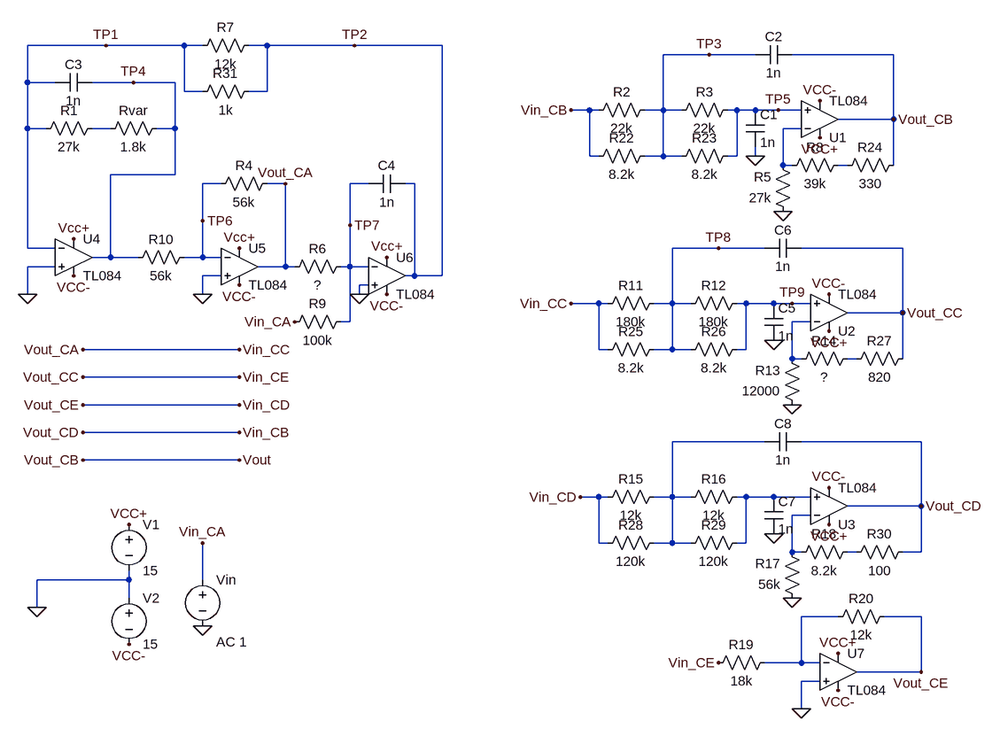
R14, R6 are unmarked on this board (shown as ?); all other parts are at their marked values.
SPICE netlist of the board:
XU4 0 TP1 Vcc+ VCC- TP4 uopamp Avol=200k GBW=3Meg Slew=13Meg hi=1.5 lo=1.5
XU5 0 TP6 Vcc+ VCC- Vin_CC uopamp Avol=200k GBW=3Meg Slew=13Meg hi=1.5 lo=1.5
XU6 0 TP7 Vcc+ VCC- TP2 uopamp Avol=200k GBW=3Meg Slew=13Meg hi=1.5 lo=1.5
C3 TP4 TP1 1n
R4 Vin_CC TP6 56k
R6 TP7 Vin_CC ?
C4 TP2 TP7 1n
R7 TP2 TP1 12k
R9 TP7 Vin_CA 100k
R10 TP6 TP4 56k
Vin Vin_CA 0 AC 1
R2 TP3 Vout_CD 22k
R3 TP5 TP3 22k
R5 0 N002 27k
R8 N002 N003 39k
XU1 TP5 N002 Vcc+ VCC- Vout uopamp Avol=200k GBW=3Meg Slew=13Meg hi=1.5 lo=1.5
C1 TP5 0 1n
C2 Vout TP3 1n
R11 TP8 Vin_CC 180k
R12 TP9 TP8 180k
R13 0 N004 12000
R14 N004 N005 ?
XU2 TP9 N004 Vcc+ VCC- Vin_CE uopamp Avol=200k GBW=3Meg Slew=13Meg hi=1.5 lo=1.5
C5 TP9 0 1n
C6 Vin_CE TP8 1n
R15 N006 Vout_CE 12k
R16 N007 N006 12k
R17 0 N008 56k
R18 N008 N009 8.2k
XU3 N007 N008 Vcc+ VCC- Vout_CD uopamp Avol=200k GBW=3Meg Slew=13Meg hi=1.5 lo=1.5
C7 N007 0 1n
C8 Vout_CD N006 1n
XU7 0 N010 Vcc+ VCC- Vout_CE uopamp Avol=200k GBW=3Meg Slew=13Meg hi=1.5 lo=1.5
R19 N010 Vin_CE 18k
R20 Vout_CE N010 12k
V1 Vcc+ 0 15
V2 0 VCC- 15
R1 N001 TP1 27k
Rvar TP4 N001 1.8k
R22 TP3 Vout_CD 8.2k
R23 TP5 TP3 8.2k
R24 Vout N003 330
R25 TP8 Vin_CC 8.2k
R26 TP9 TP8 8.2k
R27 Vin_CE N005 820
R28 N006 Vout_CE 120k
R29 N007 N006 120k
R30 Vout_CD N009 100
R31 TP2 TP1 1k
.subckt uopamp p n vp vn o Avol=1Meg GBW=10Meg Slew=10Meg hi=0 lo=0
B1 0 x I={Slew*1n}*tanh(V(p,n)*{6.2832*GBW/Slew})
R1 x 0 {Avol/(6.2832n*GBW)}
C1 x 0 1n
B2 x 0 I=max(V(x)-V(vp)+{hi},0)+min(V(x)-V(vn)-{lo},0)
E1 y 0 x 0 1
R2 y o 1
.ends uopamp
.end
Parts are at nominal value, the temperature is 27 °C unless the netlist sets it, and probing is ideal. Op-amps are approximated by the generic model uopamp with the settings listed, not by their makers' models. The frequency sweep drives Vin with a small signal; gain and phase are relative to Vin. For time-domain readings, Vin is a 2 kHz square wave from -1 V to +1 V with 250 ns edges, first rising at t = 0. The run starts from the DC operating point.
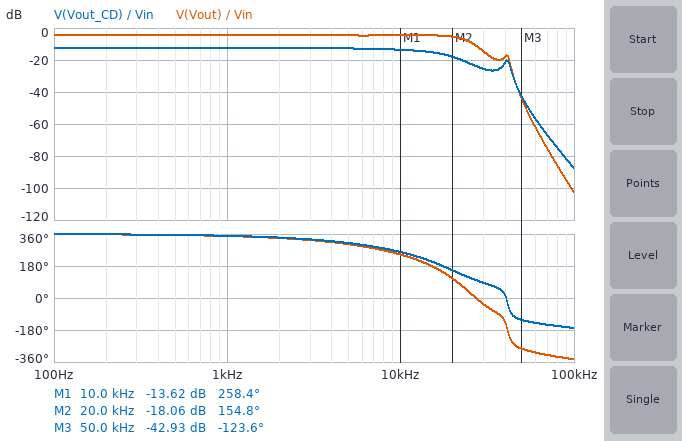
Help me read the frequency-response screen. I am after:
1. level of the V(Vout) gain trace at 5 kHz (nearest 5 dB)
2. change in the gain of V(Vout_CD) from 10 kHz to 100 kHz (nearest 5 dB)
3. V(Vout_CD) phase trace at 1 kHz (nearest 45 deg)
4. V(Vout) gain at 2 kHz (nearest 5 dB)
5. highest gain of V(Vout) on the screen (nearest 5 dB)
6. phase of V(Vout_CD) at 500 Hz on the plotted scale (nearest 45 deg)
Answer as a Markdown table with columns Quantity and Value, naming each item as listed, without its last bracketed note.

| Quantity | Value |
|---|---|
| level of the V(Vout) gain trace at 5 kHz | -5 dB |
| change in the gain of V(Vout_CD) from 10 kHz to 100 kHz | -75 dB |
| V(Vout_CD) phase trace at 1 kHz | 360 deg |
| V(Vout) gain at 2 kHz | -5 dB |
| highest gain of V(Vout) on the screen | -5 dB |
| phase of V(Vout_CD) at 500 Hz on the plotted scale | 360 deg |
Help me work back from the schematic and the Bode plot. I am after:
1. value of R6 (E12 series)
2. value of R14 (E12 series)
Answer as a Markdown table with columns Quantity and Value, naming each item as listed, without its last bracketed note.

| Quantity | Value |
|---|---|
| value of R6 | 15 kΩ |
| value of R14 | 12 kΩ |
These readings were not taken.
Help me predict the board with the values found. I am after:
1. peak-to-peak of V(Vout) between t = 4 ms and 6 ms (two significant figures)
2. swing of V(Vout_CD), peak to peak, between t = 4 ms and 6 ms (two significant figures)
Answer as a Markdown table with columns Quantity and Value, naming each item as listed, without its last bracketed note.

| Quantity | Value |
|---|---|
| peak-to-peak of V(Vout) between t = 4 ms and 6 ms | 1.5 V |
| swing of V(Vout_CD), peak to peak, between t = 4 ms and 6 ms | 510 mV |
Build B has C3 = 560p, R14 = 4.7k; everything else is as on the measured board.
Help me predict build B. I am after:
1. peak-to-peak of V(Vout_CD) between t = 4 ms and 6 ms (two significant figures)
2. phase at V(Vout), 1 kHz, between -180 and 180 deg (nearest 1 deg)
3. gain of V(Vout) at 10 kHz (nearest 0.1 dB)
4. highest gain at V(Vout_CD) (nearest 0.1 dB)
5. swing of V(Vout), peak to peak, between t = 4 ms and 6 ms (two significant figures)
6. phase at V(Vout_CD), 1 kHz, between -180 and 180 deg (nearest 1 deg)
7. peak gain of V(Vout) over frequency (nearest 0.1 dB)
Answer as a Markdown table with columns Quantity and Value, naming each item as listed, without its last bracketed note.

| Quantity | Value |
|---|---|
| peak-to-peak of V(Vout_CD) between t = 4 ms and 6 ms | 340 mV |
| phase at V(Vout), 1 kHz, between -180 and 180 deg | -13 deg |
| gain of V(Vout) at 10 kHz | -9.6 dB |
| highest gain at V(Vout_CD) | -15.5 dB |
| swing of V(Vout), peak to peak, between t = 4 ms and 6 ms | 840 mV |
| phase at V(Vout_CD), 1 kHz, between -180 and 180 deg | -12 deg |
| peak gain of V(Vout) over frequency | -7.7 dB |
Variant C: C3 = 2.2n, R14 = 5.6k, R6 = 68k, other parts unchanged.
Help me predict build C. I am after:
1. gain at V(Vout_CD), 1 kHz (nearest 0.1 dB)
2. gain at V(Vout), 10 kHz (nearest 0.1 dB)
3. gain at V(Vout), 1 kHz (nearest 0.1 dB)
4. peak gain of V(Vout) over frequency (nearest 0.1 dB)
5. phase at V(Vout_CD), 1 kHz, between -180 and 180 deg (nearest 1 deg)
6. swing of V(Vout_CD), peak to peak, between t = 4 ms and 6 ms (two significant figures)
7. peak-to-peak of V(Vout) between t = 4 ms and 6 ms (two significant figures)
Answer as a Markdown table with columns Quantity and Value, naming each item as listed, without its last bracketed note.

| Quantity | Value |
|---|---|
| gain at V(Vout_CD), 1 kHz | -1.9 dB |
| gain at V(Vout), 10 kHz | 10.7 dB |
| gain at V(Vout), 1 kHz | 5.9 dB |
| peak gain of V(Vout) over frequency | 18.1 dB |
| phase at V(Vout_CD), 1 kHz, between -180 and 180 deg | -12 deg |
| swing of V(Vout_CD), peak to peak, between t = 4 ms and 6 ms | 2.9 V |
| peak-to-peak of V(Vout) between t = 4 ms and 6 ms | 8.2 V |
